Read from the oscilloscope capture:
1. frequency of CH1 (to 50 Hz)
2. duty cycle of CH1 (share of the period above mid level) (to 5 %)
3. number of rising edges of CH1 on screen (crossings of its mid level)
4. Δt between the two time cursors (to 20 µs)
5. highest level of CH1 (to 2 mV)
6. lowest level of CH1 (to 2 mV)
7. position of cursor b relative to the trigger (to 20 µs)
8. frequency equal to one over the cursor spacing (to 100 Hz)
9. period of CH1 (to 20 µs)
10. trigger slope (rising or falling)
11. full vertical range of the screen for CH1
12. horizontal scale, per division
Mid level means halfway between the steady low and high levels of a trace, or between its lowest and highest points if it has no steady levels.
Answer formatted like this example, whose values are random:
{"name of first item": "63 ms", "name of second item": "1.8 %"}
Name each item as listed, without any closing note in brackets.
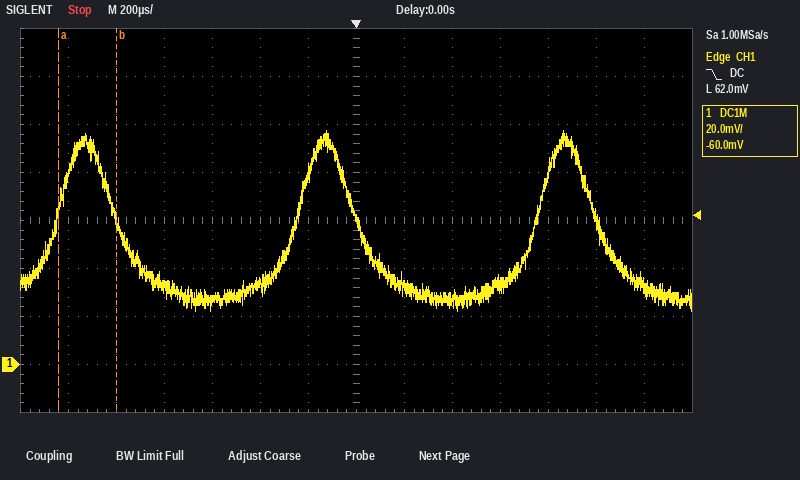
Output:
{"frequency of CH1": "1.00 kHz", "duty cycle of CH1 (share of the period above mid level)": "25 %", "number of rising edges of CH1 on screen": "3", "Δt between the two time cursors": "240 µs", "highest level of CH1": "98 mV", "lowest level of CH1": "22 mV", "position of cursor b relative to the trigger": "-1.00 ms", "frequency equal to one over the cursor spacing": "4.2 kHz", "period of CH1": "1.00 ms", "trigger slope": "falling", "full vertical range of the screen for CH1": "160 mV", "horizontal scale, per division": "200 µs"}
